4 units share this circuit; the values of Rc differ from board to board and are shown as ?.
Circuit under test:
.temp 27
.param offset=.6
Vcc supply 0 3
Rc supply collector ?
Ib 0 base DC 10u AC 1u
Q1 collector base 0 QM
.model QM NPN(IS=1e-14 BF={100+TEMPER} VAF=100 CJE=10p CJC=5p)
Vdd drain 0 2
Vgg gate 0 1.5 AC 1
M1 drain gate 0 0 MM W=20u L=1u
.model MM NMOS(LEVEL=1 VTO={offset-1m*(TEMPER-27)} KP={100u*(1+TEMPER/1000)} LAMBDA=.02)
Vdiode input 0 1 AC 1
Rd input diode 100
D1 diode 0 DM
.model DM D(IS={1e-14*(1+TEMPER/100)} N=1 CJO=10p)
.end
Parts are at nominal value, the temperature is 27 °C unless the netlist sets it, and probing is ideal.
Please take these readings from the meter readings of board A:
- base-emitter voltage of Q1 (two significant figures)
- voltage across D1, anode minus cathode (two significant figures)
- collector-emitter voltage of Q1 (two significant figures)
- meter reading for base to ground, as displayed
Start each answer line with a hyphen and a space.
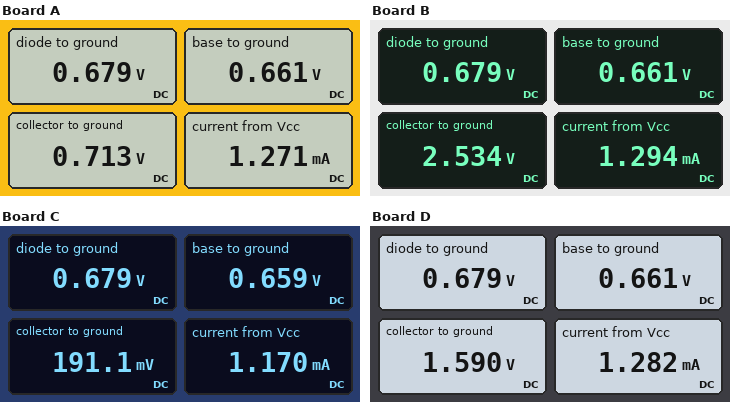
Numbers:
- 660 mV
- 680 mV
- 710 mV
- 0.661 V
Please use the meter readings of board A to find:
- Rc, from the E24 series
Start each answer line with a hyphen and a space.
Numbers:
- 1.8 kΩ
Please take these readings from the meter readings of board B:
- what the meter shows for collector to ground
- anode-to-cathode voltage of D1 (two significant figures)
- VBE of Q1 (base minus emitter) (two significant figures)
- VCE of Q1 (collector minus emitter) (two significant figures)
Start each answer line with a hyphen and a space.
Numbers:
- 2.534 V
- 680 mV
- 660 mV
- 2.5 V
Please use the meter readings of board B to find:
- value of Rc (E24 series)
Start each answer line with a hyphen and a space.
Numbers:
- 360 Ω
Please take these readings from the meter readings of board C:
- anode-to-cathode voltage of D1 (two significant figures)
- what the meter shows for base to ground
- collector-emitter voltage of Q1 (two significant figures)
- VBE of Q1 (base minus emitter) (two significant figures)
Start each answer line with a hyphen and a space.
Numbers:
- 680 mV
- 0.659 V
- 190 mV
- 660 mV
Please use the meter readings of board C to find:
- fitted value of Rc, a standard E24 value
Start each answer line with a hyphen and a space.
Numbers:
- 2.4 kΩ
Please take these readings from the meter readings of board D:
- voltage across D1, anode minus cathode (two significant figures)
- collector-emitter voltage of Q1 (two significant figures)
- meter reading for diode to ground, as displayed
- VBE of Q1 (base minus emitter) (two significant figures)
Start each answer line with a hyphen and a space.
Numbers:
- 680 mV
- 1.6 V
- 0.679 V
- 660 mV
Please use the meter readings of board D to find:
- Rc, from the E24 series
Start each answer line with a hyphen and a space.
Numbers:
- 1.1 kΩ
